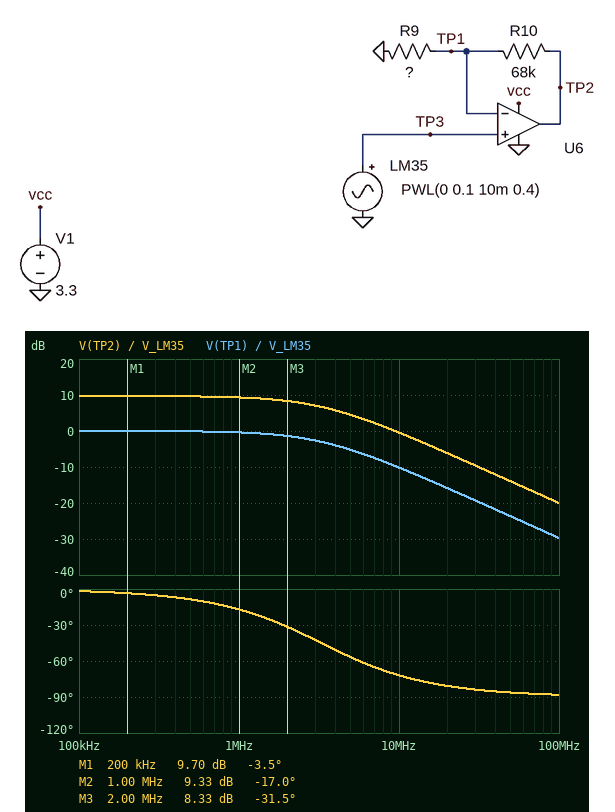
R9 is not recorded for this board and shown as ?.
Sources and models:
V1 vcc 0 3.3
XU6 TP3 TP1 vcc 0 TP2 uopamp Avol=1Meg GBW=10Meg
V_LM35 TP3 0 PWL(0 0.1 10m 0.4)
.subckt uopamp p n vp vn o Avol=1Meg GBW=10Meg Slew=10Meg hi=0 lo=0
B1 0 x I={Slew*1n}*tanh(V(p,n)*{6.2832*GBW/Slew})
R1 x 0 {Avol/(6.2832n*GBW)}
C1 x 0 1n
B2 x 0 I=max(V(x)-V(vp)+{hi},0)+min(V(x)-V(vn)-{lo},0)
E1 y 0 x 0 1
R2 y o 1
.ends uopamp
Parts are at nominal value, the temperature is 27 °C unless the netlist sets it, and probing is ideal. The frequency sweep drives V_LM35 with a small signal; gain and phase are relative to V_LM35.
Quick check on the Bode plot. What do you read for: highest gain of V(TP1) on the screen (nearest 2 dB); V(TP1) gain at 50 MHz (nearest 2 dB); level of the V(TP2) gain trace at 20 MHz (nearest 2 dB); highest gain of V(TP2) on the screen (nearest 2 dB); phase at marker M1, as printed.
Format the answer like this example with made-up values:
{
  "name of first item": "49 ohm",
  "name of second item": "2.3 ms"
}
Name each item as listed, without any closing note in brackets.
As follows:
{
  "highest gain of V(TP1) on the screen": "0 dB",
  "V(TP1) gain at 50 MHz": "-24 dB",
  "level of the V(TP2) gain trace at 20 MHz": "-6 dB",
  "highest gain of V(TP2) on the screen": "10 dB",
  "phase at marker M1, as printed": "-3.5 deg"
}
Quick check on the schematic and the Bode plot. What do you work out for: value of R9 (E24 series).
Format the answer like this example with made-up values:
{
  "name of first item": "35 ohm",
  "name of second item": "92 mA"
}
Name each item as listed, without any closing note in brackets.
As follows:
{
  "value of R9": "33 kΩ"
}
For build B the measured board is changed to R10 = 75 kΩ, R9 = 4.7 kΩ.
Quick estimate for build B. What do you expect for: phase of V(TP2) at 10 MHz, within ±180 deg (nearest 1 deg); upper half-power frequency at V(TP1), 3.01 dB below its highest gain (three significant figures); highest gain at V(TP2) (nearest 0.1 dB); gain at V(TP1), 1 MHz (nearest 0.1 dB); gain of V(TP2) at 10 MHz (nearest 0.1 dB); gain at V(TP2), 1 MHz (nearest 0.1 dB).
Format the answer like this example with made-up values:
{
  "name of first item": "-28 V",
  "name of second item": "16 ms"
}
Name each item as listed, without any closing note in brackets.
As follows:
{
  "phase of V(TP2) at 10 MHz, within ±180 deg": "-87 deg",
  "upper half-power frequency at V(TP1), 3.01 dB below its highest gain": "590 kHz",
  "highest gain at V(TP2)": "24.6 dB",
  "gain at V(TP1), 1 MHz": "-5.9 dB",
  "gain of V(TP2) at 10 MHz": "0 dB",
  "gain at V(TP2), 1 MHz": "18.7 dB"
}
